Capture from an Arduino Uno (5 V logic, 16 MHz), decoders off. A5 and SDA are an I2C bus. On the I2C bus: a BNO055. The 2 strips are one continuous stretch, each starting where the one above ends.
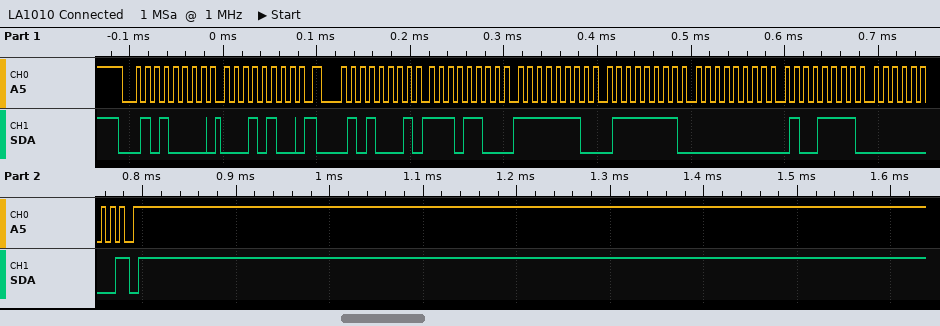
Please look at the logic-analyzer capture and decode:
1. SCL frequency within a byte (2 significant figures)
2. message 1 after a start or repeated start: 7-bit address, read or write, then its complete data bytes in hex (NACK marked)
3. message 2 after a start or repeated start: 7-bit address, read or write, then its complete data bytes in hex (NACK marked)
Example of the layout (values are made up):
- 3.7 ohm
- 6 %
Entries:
- 100 kHz
- 0x28 write: 14
- 0x28 read: EC FE 7F 00 4F 00 NACK
